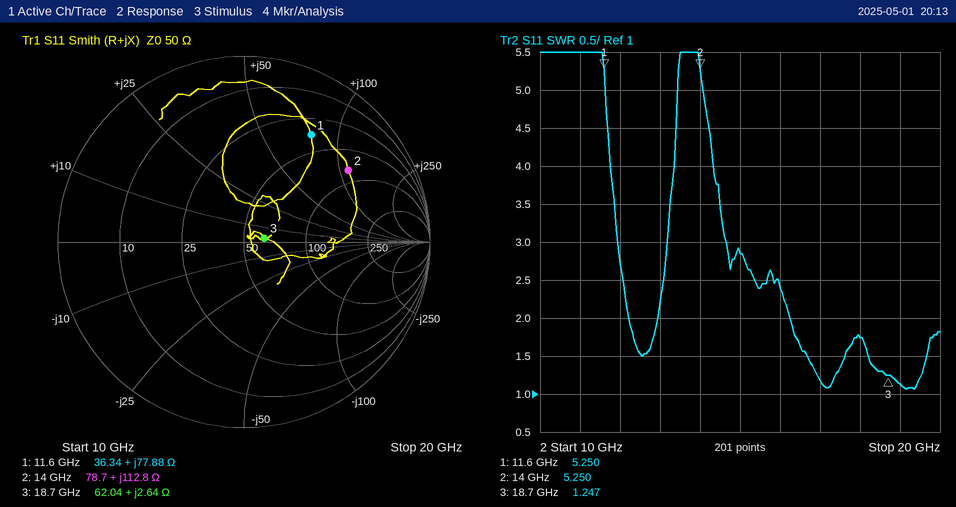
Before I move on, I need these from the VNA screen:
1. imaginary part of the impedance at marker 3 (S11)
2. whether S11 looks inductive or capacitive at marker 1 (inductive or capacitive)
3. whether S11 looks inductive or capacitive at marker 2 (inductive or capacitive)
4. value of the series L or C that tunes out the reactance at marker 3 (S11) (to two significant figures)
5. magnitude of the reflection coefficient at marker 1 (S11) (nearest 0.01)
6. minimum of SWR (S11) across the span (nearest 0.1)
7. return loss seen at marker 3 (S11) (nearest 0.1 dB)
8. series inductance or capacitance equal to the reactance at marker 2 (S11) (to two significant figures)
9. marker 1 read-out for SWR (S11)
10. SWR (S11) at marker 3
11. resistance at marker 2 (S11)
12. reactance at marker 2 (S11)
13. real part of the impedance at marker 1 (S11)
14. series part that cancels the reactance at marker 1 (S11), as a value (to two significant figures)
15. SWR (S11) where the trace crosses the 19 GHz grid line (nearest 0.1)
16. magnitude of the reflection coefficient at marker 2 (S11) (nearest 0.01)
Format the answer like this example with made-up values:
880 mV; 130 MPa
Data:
+2.64 Ω; inductive; inductive; 3.2 pF; 0.68; 1.1; 19.2 dB; 1.3 nH; 5.250; 1.247; 78.7 Ω; +112.8 Ω; 36.34 Ω; 180 fF; 1.1; 0.68
